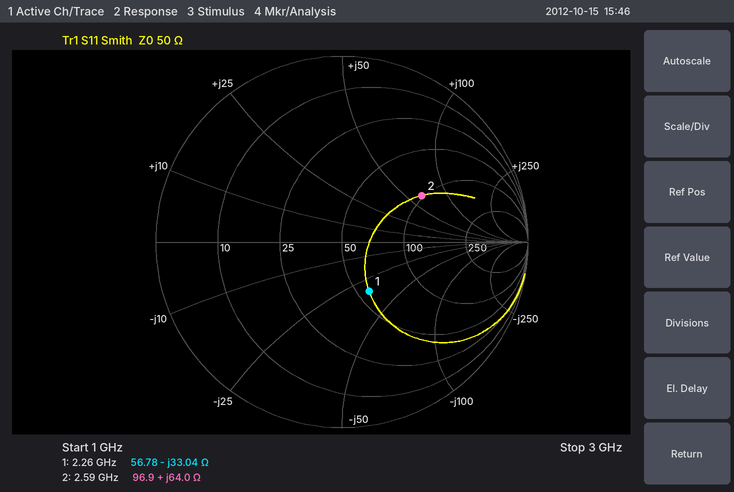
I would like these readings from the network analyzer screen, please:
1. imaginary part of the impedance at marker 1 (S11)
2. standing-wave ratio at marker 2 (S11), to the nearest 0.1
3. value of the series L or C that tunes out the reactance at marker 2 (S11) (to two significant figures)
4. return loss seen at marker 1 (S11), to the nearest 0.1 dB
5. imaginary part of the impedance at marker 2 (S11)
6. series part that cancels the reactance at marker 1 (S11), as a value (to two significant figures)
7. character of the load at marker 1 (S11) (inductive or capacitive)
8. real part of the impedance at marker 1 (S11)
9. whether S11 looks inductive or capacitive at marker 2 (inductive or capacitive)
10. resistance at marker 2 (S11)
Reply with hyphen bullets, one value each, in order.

- -33.04 Ω
- 3.0
- 960 fF
- 10.4 dB
- +64.0 Ω
- 2.3 nH
- capacitive
- 56.78 Ω
- inductive
- 96.9 Ω
